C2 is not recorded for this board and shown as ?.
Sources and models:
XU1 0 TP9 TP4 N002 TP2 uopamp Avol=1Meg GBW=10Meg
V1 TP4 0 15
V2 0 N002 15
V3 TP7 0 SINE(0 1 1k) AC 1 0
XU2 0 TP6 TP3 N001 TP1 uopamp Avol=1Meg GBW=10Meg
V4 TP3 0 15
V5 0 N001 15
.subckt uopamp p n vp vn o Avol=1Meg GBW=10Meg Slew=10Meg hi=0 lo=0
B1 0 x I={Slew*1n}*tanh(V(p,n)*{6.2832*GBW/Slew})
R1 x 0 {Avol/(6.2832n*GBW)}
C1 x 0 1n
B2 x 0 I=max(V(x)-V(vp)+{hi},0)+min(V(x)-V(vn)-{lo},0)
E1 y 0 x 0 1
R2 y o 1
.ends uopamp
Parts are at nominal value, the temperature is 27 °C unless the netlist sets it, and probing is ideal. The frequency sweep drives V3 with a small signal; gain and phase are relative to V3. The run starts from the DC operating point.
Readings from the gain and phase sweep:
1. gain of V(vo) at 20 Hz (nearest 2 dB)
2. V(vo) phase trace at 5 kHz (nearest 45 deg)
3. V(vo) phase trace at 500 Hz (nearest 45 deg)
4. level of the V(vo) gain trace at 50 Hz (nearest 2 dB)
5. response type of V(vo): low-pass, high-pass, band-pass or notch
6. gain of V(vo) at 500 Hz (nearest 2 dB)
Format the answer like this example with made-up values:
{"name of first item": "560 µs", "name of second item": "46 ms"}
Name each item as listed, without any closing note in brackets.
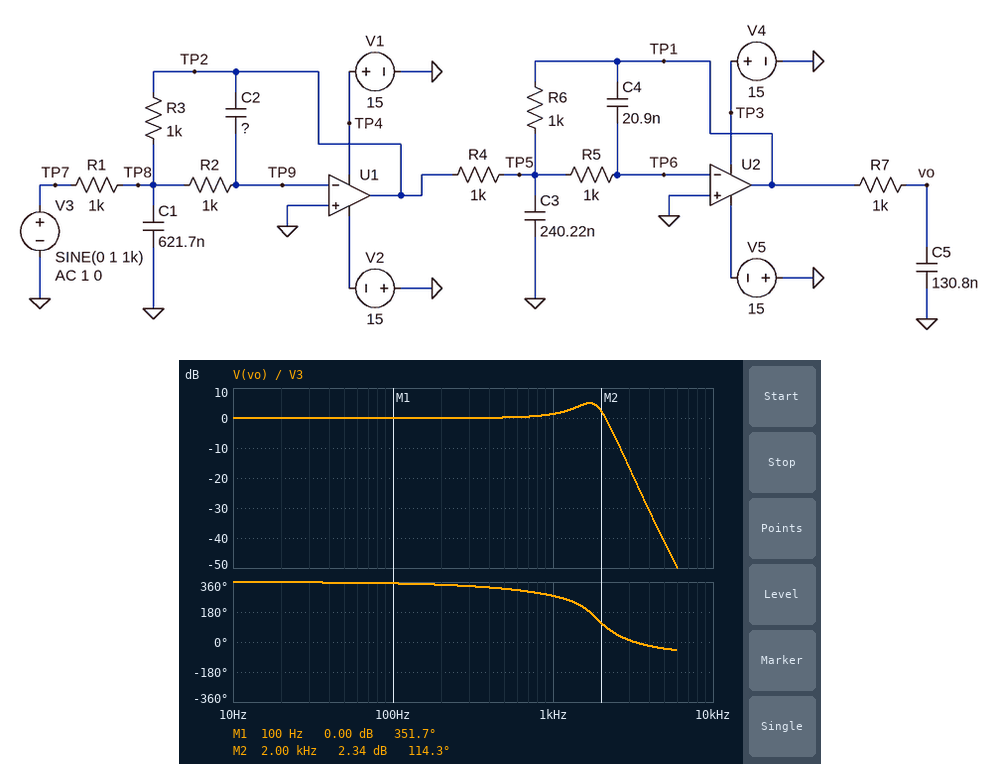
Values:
{"gain of V(vo) at 20 Hz": "0 dB", "V(vo) phase trace at 5 kHz": "-45 deg", "V(vo) phase trace at 500 Hz": "315 deg", "level of the V(vo) gain trace at 50 Hz": "0 dB", "response type of V(vo): low-pass, high-pass, band-pass or notch": "low-pass", "gain of V(vo) at 500 Hz": "0 dB"}
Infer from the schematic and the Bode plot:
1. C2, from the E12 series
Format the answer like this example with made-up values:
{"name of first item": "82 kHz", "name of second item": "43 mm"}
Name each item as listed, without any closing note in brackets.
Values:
{"C2, from the E12 series": "12 nF"}
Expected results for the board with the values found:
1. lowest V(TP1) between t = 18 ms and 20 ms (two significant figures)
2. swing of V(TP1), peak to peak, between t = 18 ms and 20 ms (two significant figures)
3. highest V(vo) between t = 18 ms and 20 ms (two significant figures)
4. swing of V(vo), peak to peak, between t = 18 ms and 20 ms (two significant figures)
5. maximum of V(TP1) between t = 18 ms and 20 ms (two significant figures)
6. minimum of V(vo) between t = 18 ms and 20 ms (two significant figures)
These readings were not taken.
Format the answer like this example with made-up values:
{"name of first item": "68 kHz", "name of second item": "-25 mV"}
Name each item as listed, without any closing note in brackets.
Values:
{"lowest V(TP1) between t = 18 ms and 20 ms": "-1.5 V", "swing of V(TP1), peak to peak, between t = 18 ms and 20 ms": "3.0 V", "highest V(vo) between t = 18 ms and 20 ms": "1.2 V", "swing of V(vo), peak to peak, between t = 18 ms and 20 ms": "2.3 V", "maximum of V(TP1) between t = 18 ms and 20 ms": "1.5 V", "minimum of V(vo) between t = 18 ms and 20 ms": "-1.2 V"}
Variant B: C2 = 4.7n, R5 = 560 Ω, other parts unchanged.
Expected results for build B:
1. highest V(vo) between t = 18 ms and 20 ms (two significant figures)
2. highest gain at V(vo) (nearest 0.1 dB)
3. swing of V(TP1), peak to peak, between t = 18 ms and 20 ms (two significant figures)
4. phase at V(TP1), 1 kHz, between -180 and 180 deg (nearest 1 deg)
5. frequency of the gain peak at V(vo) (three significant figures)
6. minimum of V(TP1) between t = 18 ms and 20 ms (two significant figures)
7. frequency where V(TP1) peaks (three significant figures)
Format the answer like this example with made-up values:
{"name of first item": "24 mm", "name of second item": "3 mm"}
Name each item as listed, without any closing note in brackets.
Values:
{"highest V(vo) between t = 18 ms and 20 ms": "930 mV", "highest gain at V(vo)": "5.6 dB", "swing of V(TP1), peak to peak, between t = 18 ms and 20 ms": "2.4 V", "phase at V(TP1), 1 kHz, between -180 and 180 deg": "-23 deg", "frequency of the gain peak at V(vo)": "2.80 kHz", "minimum of V(TP1) between t = 18 ms and 20 ms": "-1.2 V", "frequency where V(TP1) peaks": "2.85 kHz"}
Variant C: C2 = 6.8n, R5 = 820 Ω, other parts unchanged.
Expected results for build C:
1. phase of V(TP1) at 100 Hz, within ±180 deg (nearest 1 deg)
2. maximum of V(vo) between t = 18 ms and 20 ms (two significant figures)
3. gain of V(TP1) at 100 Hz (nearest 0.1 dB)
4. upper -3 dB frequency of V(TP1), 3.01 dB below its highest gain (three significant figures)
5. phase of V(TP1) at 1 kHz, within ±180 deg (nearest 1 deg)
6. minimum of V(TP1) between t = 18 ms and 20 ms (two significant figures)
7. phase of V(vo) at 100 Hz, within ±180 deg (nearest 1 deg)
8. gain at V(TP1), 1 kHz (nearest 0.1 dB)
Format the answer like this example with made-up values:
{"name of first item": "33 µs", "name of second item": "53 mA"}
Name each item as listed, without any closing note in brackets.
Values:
{"phase of V(TP1) at 100 Hz, within ±180 deg": "-3 deg", "maximum of V(vo) between t = 18 ms and 20 ms": "1.0 V", "gain of V(TP1) at 100 Hz": "0 dB", "upper -3 dB frequency of V(TP1), 3.01 dB below its highest gain": "2.66 kHz", "phase of V(TP1) at 1 kHz, within ±180 deg": "-31 deg", "minimum of V(TP1) between t = 18 ms and 20 ms": "-1.3 V", "phase of V(vo) at 100 Hz, within ±180 deg": "-7 deg", "gain at V(TP1), 1 kHz": "2.3 dB"}
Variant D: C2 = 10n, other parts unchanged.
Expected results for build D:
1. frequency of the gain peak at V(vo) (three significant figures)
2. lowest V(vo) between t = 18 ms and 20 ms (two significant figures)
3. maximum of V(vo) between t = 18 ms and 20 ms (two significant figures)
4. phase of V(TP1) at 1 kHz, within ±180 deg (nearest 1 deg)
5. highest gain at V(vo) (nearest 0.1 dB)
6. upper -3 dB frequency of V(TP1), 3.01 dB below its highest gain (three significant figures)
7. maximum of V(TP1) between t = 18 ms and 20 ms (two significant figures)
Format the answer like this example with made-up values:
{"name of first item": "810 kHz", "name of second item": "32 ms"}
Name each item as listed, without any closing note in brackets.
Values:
{"frequency of the gain peak at V(vo)": "1.86 kHz", "lowest V(vo) between t = 18 ms and 20 ms": "-1.1 V", "maximum of V(vo) between t = 18 ms and 20 ms": "1.1 V", "phase of V(TP1) at 1 kHz, within ±180 deg": "-40 deg", "highest gain at V(vo)": "5.1 dB", "upper -3 dB frequency of V(TP1), 3.01 dB below its highest gain": "2.24 kHz", "maximum of V(TP1) between t = 18 ms and 20 ms": "1.4 V"}
